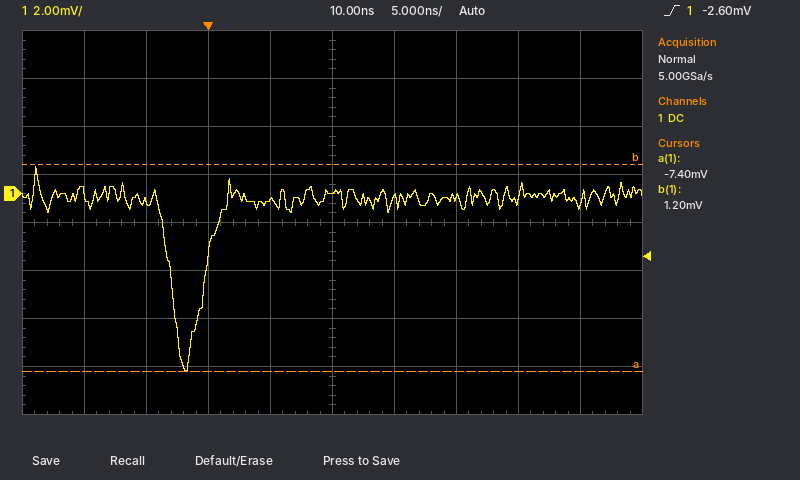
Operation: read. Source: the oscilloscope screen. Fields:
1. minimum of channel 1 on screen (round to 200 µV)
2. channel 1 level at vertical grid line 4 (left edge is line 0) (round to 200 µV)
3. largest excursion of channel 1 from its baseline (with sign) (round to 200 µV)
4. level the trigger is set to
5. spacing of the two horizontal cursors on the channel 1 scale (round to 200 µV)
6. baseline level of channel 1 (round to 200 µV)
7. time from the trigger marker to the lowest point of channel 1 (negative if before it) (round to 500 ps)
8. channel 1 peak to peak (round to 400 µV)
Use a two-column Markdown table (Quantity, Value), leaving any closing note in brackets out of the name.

| Quantity | Value |
|---|---|
| minimum of channel 1 on screen | -7.4 mV |
| channel 1 level at vertical grid line 4 (left edge is line 0) | -200 µV |
| largest excursion of channel 1 from its baseline (with sign) | -7.2 mV |
| level the trigger is set to | -2.60 mV |
| spacing of the two horizontal cursors on the channel 1 scale | 8.6 mV |
| baseline level of channel 1 | -200 µV |
| time from the trigger marker to the lowest point of channel 1 (negative if before it) | -2.0 ns |
| channel 1 peak to peak | 8.4 mV |
